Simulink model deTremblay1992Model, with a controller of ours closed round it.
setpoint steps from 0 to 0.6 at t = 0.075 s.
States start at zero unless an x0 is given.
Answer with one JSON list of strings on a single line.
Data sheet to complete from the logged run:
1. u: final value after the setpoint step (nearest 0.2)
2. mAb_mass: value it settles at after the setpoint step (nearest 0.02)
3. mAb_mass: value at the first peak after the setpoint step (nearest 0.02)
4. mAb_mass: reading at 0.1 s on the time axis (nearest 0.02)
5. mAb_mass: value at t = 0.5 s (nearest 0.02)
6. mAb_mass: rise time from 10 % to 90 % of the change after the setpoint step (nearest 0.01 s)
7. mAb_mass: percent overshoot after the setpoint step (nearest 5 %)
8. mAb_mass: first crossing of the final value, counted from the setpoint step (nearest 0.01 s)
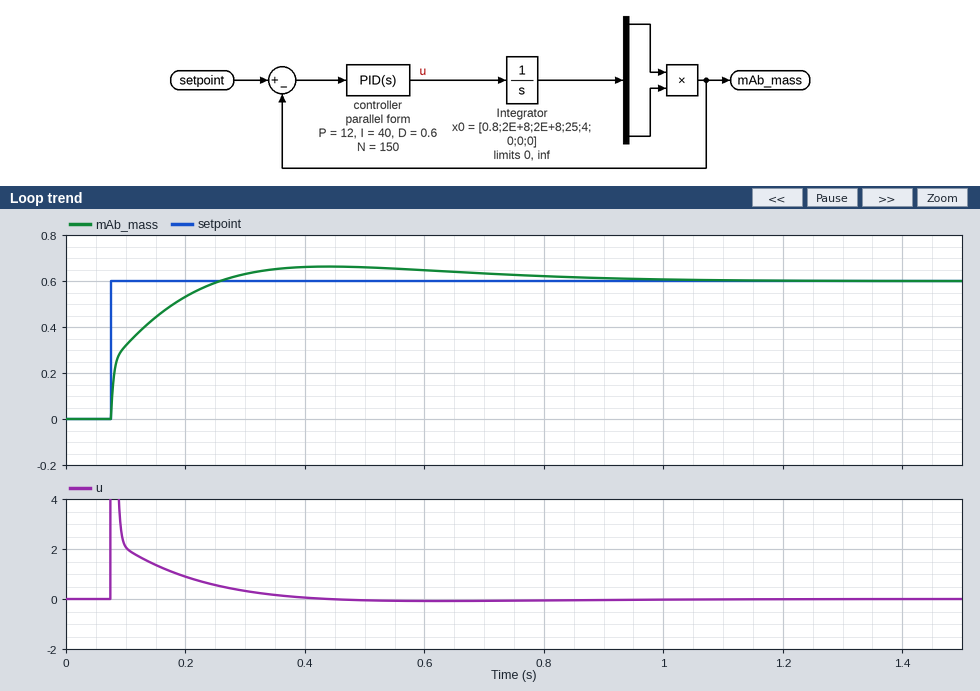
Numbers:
["0.0", "0.60", "0.66", "0.32", "0.66", "0.13 s", "10 %", "0.18 s"]
